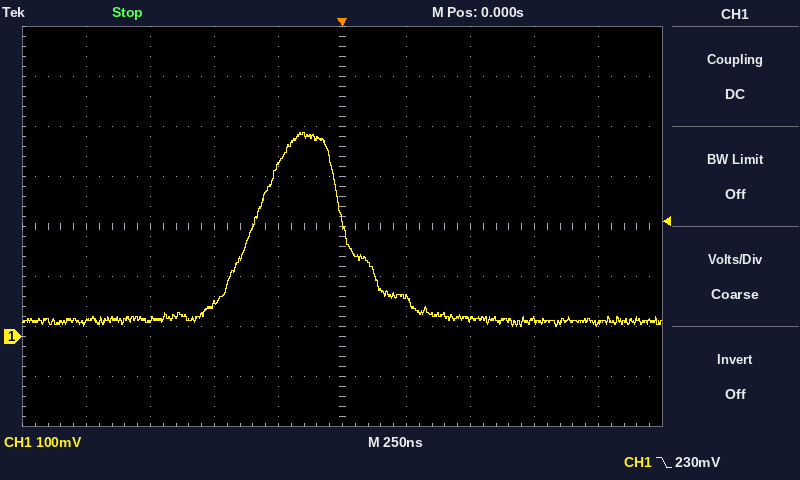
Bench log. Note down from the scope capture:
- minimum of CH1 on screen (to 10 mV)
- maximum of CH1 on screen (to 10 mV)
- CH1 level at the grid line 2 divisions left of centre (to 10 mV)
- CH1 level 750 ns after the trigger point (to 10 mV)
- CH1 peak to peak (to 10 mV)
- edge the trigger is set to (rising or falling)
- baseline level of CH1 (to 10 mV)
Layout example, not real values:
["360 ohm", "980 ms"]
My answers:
["20 mV", "410 mV", "60 mV", "30 mV", "390 mV", "falling", "30 mV"]
